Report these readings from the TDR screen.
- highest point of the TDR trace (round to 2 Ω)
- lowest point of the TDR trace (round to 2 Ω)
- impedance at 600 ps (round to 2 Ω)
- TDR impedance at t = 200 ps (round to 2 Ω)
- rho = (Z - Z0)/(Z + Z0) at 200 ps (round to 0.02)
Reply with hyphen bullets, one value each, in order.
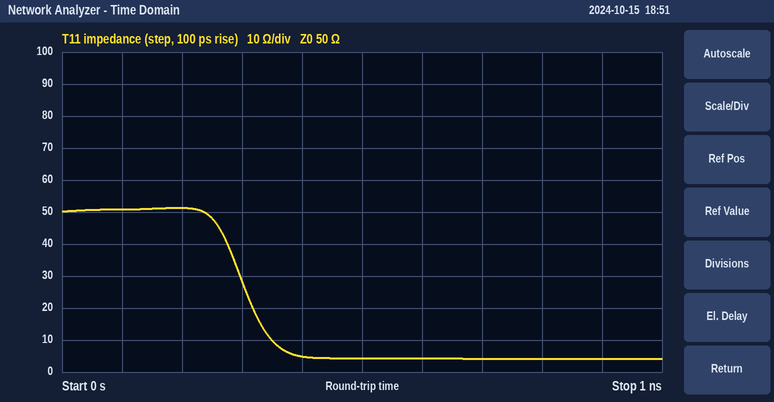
- 52 Ω
- 4 Ω
- 4 Ω
- 52 Ω
- +0.02
